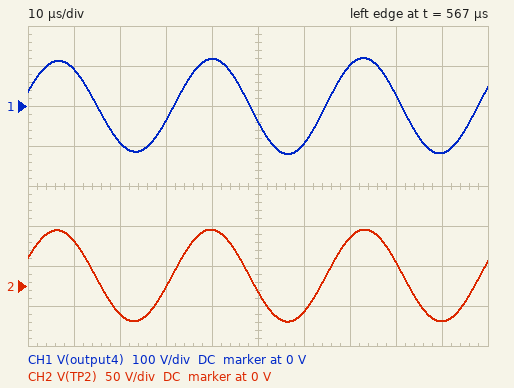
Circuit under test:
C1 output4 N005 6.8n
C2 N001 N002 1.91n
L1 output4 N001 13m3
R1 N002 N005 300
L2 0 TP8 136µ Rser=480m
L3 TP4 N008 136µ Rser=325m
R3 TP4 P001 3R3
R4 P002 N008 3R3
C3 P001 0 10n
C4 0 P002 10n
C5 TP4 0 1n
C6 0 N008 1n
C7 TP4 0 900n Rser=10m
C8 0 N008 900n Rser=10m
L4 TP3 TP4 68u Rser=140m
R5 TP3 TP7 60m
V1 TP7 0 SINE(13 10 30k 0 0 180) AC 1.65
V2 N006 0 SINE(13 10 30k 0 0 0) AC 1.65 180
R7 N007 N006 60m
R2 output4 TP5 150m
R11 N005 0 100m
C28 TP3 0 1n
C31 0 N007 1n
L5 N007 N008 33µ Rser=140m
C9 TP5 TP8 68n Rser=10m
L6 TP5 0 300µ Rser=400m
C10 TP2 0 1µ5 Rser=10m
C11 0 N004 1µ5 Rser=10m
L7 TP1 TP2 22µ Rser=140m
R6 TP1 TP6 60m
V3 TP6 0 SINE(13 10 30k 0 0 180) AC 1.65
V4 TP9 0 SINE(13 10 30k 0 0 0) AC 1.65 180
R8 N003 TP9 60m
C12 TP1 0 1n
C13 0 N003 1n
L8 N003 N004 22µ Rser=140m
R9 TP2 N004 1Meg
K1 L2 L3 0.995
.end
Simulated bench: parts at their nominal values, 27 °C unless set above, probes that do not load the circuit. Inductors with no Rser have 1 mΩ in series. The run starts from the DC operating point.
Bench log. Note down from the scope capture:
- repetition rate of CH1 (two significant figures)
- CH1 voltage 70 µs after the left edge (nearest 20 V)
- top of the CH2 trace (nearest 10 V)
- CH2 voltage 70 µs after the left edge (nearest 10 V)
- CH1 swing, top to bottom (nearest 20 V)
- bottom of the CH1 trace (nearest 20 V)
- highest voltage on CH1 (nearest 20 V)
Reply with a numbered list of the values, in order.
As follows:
1. 30 kHz
2. 100 V
3. 70 V
4. 60 V
5. 240 V
6. -120 V
7. 120 V
